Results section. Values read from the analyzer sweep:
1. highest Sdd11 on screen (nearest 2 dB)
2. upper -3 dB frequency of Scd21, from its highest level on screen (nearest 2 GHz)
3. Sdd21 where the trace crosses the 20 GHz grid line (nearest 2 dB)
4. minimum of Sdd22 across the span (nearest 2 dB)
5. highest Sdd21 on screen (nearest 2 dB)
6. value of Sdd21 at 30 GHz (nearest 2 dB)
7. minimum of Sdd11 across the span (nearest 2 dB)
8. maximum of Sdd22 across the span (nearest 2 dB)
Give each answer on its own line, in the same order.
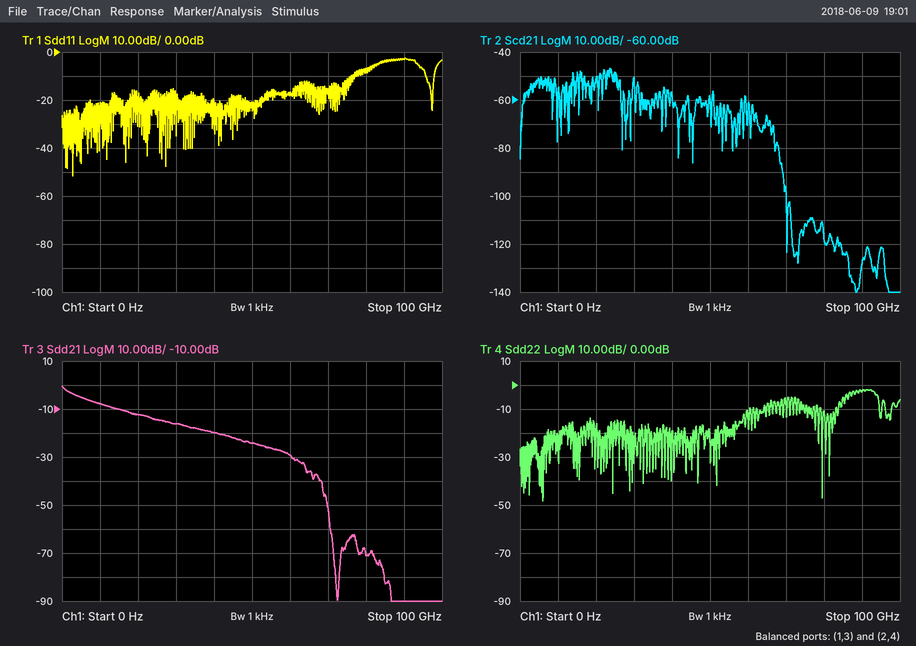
-2 dB
24 GHz
-12 dB
-48 dB
0 dB
-16 dB
-52 dB
-2 dB
